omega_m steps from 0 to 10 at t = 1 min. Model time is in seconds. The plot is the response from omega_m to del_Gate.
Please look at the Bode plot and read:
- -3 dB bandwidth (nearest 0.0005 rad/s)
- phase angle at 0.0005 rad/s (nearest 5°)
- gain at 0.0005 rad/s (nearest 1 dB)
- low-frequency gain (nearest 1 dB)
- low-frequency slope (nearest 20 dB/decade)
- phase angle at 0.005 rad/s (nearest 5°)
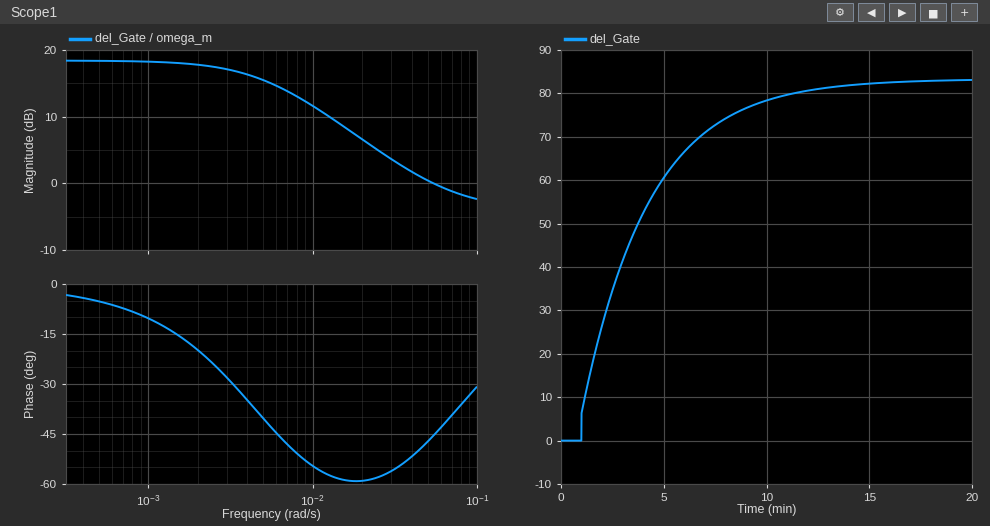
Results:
0.0050 rad/s
-5°
18 dB
18 dB
0 dB/decade
-40°
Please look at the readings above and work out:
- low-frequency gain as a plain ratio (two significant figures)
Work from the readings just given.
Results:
7.9
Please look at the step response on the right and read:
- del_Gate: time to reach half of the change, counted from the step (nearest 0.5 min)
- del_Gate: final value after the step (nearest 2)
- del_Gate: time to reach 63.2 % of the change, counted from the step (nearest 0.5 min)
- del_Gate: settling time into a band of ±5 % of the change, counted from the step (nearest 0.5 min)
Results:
2.0 min
84
3.0 min
9.5 min
